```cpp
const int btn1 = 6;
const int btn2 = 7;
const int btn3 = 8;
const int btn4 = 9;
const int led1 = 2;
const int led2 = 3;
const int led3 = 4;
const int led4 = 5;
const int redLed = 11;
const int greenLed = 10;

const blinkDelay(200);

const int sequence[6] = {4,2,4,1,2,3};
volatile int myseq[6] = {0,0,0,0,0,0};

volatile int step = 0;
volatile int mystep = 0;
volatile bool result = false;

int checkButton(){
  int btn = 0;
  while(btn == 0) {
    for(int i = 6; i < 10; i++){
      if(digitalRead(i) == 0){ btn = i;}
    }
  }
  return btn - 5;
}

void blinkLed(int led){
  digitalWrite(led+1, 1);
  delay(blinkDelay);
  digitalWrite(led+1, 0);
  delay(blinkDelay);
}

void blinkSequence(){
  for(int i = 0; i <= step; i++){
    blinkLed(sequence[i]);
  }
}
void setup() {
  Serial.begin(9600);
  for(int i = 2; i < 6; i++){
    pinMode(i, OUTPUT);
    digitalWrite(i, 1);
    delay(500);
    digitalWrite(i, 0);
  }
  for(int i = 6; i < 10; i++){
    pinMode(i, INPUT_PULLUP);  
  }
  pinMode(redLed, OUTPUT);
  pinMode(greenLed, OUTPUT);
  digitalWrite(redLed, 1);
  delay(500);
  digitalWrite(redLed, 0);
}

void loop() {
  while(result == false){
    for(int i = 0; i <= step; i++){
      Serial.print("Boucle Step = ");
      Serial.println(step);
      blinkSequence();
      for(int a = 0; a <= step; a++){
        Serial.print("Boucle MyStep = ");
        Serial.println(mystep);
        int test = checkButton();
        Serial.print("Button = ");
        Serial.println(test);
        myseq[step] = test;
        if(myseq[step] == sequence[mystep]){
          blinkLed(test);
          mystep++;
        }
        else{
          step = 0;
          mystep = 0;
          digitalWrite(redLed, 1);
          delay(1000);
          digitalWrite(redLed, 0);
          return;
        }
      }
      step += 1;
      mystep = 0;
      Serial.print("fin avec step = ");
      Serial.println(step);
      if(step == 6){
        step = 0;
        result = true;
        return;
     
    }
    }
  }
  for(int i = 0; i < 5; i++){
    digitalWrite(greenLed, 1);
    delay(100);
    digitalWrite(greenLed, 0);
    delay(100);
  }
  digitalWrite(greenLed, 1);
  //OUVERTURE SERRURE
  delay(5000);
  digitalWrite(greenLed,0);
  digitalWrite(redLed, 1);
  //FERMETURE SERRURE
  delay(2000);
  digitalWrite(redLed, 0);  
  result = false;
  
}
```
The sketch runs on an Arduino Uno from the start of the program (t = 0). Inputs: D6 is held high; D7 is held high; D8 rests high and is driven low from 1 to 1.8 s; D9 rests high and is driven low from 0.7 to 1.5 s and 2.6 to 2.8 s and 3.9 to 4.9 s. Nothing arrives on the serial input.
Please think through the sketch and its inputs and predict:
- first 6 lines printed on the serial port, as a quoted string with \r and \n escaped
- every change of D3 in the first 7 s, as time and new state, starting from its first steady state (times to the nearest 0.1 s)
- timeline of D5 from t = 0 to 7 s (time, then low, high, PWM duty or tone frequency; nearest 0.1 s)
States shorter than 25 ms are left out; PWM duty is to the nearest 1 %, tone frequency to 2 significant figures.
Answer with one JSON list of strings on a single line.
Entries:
["\"Boucle Step = 0\\r\\nBoucle MyStep = 0\\r\\nButton = 4\\r\\nfin avec step = 1\\r\\nBoucle Step = 1\\r\\nBoucle MyStep = 0\\r\\n\"", "0.5 s high; 1 s low; 4.7 s high; 4.9 s low", "1.5 s high; 2 s low; 2.5 s high; 2.7 s low; 3.9 s high; 4.1 s low; 4.3 s high; 4.5 s low"]
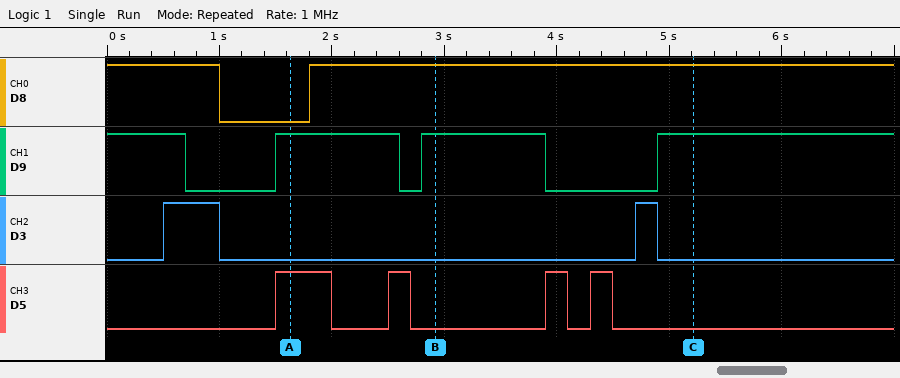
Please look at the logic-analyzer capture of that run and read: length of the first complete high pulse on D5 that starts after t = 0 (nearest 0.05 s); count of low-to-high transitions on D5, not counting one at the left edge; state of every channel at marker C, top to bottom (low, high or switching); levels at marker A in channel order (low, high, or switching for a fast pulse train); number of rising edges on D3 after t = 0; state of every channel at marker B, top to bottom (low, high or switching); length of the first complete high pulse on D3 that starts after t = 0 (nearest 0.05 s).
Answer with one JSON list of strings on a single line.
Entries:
["0.50 s", "4", "D8 high, D9 high, D3 low, D5 low", "D8 low, D9 high, D3 low, D5 high", "2", "D8 high, D9 high, D3 low, D5 low", "0.50 s"]
